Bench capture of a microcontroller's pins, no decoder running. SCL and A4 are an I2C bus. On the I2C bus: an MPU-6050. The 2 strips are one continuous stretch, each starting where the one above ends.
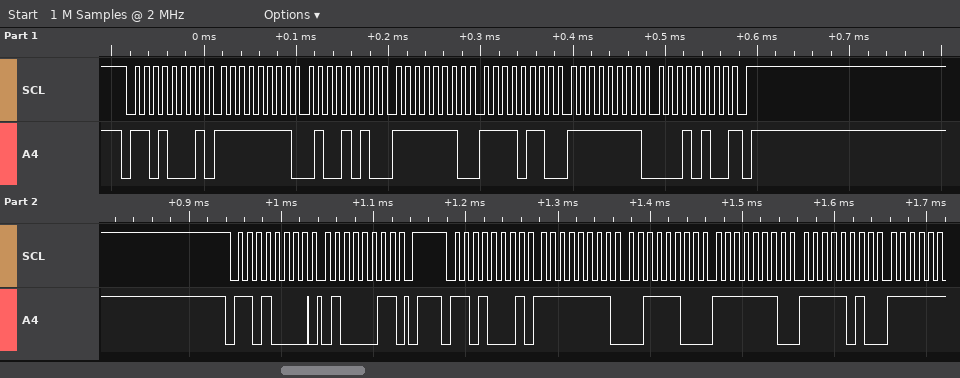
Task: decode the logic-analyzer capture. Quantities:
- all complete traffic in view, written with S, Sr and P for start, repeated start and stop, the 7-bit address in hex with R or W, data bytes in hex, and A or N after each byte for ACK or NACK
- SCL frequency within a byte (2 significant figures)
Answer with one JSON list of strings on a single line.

["S 68R A FF A 4A A FE A F6 A FF A 14 N P S 68W A 43 A P S 68R A FF A 3C A FE A FA A", "100 kHz"]
